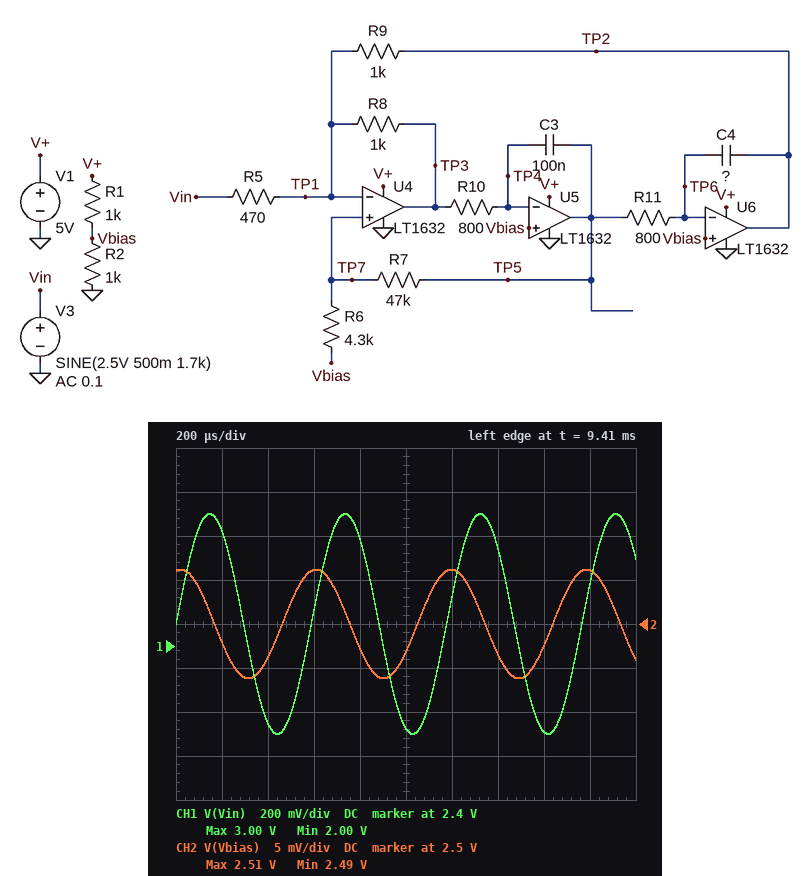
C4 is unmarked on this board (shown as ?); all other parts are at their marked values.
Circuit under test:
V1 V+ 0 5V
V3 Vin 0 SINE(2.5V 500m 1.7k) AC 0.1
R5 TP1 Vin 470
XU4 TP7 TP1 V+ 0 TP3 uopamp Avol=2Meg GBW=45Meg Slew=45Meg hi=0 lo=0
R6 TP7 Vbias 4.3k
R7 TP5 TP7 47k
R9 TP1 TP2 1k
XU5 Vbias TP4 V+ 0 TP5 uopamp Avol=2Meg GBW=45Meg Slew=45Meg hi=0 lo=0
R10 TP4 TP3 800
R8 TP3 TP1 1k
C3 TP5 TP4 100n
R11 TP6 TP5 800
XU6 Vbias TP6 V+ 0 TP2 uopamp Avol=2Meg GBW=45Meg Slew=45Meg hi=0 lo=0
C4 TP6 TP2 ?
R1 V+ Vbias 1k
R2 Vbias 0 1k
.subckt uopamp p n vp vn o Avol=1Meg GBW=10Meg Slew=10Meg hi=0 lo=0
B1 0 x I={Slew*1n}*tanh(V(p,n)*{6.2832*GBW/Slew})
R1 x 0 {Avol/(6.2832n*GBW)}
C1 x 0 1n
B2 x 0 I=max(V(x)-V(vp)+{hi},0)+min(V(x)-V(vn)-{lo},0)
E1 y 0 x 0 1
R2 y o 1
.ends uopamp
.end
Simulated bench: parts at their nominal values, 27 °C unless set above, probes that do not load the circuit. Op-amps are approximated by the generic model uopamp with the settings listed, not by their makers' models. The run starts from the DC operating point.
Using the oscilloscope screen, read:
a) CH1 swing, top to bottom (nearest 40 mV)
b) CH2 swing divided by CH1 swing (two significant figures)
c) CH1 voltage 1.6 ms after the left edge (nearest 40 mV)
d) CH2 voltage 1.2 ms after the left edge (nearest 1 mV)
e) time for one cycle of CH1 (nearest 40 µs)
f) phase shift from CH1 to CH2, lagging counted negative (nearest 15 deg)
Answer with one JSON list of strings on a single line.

["1.00 V", "0.012", "2.00 V", "2.506 V", "600 µs", "75 deg"]
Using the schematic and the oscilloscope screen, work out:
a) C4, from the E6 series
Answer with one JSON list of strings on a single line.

["47 nF"]
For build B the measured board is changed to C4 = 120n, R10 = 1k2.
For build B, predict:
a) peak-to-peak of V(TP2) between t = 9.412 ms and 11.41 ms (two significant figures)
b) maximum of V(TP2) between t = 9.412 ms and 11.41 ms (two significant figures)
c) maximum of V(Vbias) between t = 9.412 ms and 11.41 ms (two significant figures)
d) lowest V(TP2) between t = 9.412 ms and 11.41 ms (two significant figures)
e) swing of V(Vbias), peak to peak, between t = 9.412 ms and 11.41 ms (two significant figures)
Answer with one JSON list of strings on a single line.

["4.1 V", "4.5 V", "2.5 V", "470 mV", "41 mV"]
